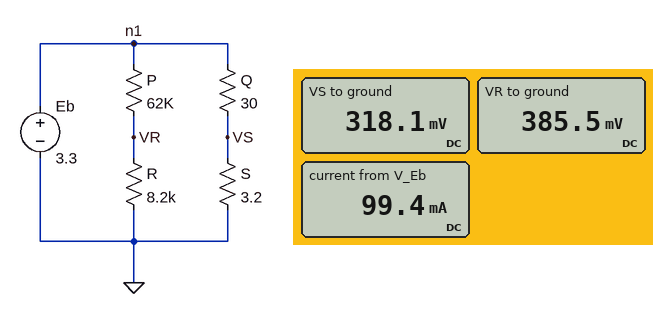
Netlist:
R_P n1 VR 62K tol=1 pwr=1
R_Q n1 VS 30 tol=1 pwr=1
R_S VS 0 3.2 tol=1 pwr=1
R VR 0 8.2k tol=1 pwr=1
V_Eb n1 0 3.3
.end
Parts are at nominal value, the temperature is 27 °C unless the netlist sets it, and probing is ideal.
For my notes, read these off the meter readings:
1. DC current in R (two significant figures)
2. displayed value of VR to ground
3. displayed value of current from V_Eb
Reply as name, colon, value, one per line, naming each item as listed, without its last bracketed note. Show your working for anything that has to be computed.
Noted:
DC current in R: (385.5 mV) / 8.2 kΩ = 47 µA
displayed value of VR to ground: 385.5 mV
displayed value of current from V_Eb: 99.4 mA
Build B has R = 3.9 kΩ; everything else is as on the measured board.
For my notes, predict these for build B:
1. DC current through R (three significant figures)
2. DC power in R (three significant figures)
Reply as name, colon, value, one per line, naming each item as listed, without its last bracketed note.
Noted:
DC current through R: 50.1 µA
DC power in R: 9.78 µW
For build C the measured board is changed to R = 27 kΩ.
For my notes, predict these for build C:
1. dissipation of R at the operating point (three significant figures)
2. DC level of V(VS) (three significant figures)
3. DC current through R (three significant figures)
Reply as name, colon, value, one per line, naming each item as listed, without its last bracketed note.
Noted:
dissipation of R at the operating point: 37.1 µW
DC level of V(VS): 318 mV
DC current through R: 37.1 µA
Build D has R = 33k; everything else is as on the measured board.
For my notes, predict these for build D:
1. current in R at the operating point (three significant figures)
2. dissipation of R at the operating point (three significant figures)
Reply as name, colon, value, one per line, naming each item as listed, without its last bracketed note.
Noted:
current in R at the operating point: 34.7 µA
dissipation of R at the operating point: 39.8 µW
